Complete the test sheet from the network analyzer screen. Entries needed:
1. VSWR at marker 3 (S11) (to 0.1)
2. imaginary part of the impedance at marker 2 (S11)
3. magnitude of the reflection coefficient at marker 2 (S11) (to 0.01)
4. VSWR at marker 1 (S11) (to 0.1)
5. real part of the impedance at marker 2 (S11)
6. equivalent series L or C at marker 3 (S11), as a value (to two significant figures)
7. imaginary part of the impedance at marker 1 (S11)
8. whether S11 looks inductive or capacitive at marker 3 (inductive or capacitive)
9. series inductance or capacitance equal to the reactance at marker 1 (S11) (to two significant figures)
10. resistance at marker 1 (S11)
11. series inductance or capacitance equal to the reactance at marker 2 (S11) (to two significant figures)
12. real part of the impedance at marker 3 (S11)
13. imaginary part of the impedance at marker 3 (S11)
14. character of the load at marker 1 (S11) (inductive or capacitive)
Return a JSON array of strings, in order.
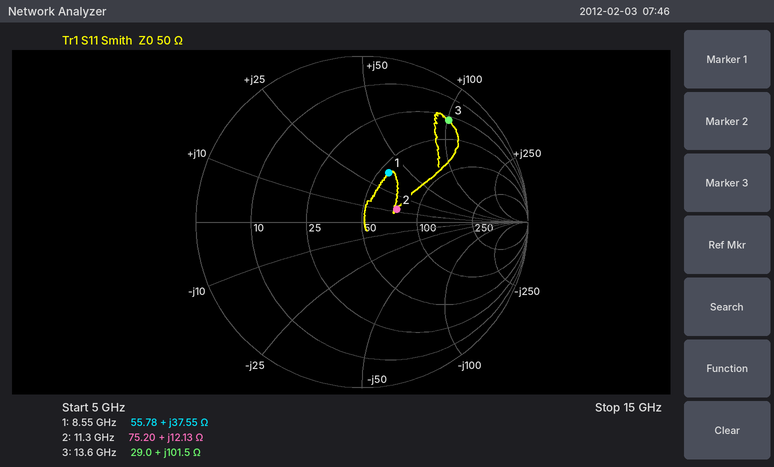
["9.3", "+12.13 Ω", "0.22", "2.0", "75.20 Ω", "1.2 nH", "+37.55 Ω", "inductive", "700 pH", "55.78 Ω", "170 pH", "29.0 Ω", "+101.5 Ω", "inductive"]
